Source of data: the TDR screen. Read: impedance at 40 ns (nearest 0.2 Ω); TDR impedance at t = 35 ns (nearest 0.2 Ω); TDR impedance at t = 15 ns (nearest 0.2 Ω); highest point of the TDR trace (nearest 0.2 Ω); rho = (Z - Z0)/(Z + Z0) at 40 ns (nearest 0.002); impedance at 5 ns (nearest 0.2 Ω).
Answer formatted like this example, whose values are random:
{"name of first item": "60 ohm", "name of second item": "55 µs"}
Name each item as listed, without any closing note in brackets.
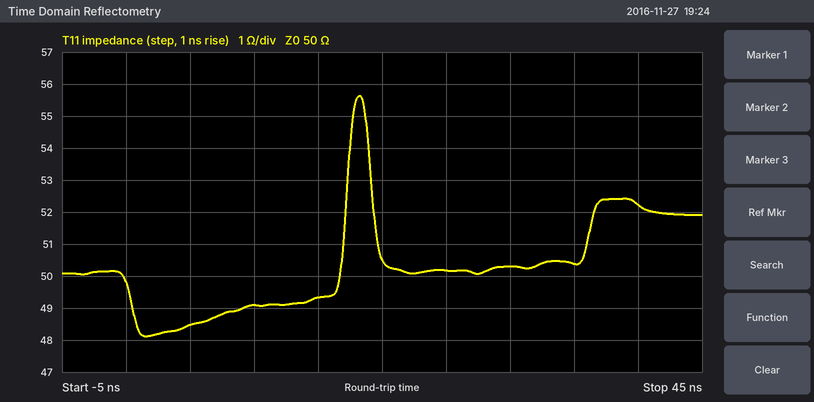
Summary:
{"impedance at 40 ns": "52.2 Ω", "TDR impedance at t = 35 ns": "50.4 Ω", "TDR impedance at t = 15 ns": "49.4 Ω", "highest point of the TDR trace": "55.6 Ω", "rho = (Z - Z0)/(Z + Z0) at 40 ns": "+0.022", "impedance at 5 ns": "48.4 Ω"}
